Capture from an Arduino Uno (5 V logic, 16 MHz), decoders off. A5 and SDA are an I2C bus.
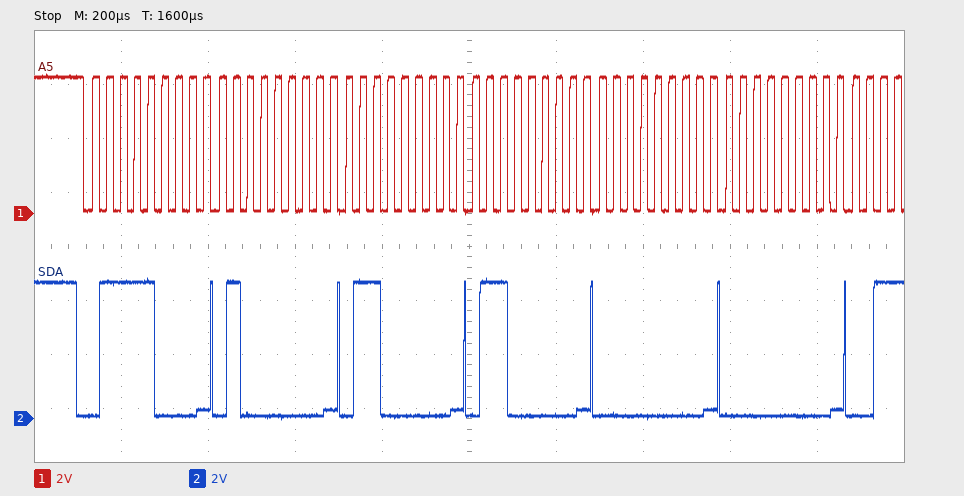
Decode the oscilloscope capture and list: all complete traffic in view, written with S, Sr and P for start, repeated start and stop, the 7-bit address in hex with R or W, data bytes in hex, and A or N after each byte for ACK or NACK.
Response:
S 3CW A 40 A 60 A 60 A 00 A 00 A
